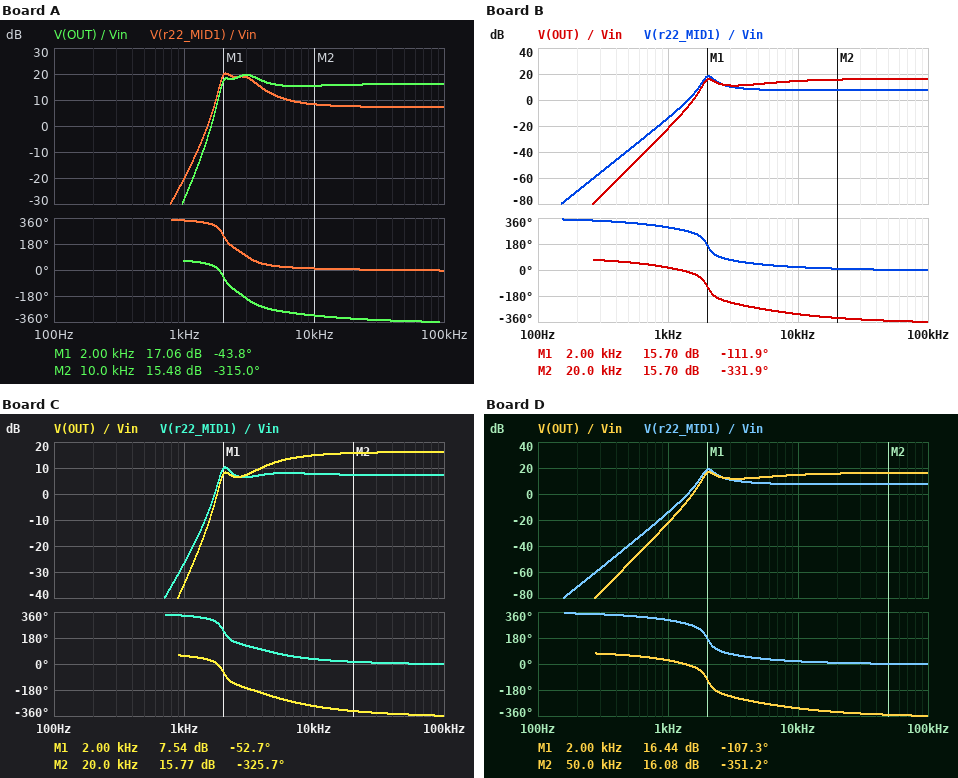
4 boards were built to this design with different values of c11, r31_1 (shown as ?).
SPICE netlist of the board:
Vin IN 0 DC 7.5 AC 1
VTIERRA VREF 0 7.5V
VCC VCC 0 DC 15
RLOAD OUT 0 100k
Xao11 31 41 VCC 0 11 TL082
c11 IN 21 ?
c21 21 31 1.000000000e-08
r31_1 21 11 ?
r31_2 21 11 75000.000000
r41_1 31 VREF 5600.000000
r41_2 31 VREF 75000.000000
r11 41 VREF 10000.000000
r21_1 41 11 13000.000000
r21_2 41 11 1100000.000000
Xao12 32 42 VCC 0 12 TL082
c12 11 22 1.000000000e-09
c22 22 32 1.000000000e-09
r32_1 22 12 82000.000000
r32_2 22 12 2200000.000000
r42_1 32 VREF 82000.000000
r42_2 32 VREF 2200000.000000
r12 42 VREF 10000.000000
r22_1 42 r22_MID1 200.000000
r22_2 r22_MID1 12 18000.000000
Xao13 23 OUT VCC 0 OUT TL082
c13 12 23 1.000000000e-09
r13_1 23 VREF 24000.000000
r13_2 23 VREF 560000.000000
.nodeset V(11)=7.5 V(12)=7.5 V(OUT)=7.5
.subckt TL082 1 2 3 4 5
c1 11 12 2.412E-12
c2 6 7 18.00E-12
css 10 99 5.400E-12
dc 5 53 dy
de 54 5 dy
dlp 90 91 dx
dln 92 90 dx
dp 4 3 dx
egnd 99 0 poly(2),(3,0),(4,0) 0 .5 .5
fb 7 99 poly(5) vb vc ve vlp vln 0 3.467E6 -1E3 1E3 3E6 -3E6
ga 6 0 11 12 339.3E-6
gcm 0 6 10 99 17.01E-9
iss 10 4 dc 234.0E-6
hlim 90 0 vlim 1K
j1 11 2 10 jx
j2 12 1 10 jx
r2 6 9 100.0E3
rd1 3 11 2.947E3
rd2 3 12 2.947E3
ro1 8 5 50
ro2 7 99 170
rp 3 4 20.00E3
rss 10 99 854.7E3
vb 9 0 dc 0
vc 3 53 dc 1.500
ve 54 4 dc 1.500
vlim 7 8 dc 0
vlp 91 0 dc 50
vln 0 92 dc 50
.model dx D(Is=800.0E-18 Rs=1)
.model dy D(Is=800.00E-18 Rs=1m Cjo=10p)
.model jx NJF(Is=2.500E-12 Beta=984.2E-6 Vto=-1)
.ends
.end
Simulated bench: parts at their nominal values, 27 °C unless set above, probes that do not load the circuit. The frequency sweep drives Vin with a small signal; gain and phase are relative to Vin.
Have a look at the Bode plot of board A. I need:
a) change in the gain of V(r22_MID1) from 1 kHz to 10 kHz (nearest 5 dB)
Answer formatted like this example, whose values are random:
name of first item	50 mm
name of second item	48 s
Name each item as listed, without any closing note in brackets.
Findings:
change in the gain of V(r22_MID1) from 1 kHz to 10 kHz	30 dB
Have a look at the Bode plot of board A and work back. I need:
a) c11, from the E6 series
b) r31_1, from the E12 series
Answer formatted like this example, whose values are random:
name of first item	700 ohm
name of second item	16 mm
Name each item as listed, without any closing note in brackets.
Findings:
c11, from the E6 series	15 nF
r31_1, from the E12 series	3.9 kΩ
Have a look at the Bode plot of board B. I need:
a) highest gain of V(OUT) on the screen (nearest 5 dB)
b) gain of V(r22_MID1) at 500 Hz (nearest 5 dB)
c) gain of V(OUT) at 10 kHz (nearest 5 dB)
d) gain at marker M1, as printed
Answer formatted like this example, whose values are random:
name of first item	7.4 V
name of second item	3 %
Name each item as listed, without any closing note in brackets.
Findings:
highest gain of V(OUT) on the screen	15 dB
gain of V(r22_MID1) at 500 Hz	-40 dB
gain of V(OUT) at 10 kHz	15 dB
gain at marker M1, as printed	15.70 dB
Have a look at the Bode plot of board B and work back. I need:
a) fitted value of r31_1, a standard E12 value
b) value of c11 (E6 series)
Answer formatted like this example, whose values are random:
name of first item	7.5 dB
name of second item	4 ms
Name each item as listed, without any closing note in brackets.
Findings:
fitted value of r31_1, a standard E12 value	8.2 kΩ
value of c11	22 nF
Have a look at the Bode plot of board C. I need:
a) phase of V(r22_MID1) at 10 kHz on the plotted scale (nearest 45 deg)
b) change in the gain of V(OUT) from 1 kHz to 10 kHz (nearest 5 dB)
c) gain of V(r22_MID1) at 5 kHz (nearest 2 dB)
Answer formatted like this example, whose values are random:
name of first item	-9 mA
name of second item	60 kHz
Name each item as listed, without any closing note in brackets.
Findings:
phase of V(r22_MID1) at 10 kHz on the plotted scale	45 deg
change in the gain of V(OUT) from 1 kHz to 10 kHz	50 dB
gain of V(r22_MID1) at 5 kHz	8 dB
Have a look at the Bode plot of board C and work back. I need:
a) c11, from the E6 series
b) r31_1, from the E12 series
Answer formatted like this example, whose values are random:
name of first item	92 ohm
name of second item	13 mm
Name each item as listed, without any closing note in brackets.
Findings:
c11, from the E6 series	3.3 nF
r31_1, from the E12 series	10 kΩ
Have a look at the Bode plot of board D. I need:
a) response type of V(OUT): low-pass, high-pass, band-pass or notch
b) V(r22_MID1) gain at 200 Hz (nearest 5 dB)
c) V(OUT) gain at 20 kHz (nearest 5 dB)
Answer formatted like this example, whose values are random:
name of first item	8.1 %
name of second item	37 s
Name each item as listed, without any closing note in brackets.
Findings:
response type of V(OUT): low-pass, high-pass, band-pass or notch	high-pass
V(r22_MID1) gain at 200 Hz	-70 dB
V(OUT) gain at 20 kHz	15 dB
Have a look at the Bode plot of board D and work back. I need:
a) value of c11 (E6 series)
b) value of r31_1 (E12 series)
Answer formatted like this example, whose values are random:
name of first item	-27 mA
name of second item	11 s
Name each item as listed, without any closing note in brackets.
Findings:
value of c11	22 nF
value of r31_1	6.8 kΩ
